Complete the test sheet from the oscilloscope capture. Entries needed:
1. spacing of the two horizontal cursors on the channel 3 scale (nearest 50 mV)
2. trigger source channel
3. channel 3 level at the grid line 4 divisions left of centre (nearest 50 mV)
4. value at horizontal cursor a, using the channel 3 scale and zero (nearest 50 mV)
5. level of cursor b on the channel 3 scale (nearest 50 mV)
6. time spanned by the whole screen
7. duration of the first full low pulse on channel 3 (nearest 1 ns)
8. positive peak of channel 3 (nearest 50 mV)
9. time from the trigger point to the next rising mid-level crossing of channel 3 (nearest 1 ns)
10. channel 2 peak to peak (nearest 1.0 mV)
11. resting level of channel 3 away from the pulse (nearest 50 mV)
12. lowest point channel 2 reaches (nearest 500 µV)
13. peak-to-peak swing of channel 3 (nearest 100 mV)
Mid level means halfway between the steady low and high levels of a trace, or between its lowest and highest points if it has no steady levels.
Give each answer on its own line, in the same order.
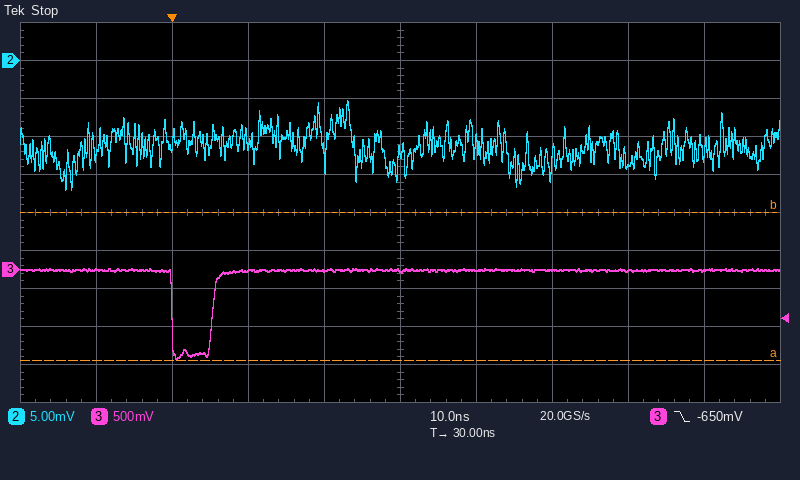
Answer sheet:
1.95 V
channel 3
0 mV
-1.20 V
750 mV
100 ns
5 ns
0 mV
5 ns
12.0 mV
0 mV
-17.0 mV
1.20 V
